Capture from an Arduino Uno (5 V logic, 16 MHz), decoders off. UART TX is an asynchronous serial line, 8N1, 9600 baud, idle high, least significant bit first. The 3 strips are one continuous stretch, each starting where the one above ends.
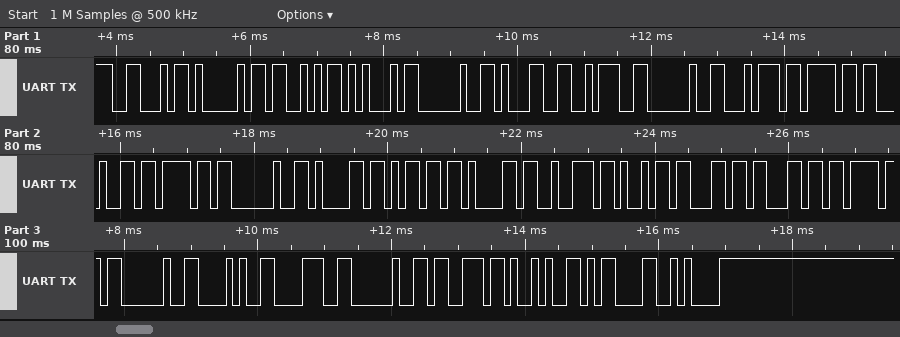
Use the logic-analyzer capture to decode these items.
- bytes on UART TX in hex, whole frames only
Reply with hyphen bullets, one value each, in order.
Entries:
- 0x46 0x41 0x53 0x45 0x20 0x31 0x3A 0x20 0x74 0x6F 0x64 0x6F 0x20 0x61 0x6D 0x61 0x72 0x69 0x6C 0x6C 0x6F 0x20 0x28 0x38 0x20 0x73 0x29 0x0D 0x0A
